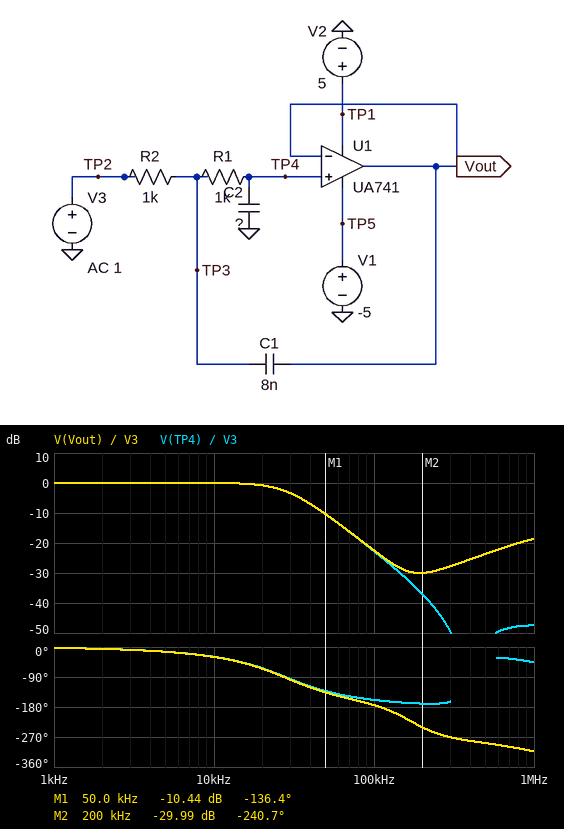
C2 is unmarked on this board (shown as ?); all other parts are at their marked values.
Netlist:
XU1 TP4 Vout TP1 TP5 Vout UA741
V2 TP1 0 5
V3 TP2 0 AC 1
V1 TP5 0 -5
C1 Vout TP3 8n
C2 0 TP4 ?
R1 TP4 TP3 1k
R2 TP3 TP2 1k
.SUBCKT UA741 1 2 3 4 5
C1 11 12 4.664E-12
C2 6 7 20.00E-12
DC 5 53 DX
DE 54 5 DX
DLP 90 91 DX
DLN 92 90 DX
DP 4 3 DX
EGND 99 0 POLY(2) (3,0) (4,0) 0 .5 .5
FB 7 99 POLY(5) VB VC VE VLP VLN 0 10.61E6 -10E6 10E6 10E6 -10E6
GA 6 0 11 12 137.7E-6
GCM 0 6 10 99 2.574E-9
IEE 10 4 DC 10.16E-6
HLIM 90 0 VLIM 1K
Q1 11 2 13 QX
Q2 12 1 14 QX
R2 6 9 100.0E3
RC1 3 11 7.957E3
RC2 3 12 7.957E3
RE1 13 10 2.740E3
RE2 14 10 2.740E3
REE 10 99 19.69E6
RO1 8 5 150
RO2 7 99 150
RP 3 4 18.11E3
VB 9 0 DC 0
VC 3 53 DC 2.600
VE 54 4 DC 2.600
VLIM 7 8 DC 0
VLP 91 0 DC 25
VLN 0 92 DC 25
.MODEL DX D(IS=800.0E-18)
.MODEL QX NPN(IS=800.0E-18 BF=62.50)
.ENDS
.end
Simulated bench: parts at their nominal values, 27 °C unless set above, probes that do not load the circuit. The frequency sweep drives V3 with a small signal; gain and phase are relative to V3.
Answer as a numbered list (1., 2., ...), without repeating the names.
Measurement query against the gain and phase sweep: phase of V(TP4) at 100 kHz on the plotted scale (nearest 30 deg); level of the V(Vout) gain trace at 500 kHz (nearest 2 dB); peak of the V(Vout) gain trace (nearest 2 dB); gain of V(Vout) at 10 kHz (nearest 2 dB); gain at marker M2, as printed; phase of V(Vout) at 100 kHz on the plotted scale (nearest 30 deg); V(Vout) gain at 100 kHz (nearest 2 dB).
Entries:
1. -150 deg
2. -24 dB
3. 0 dB
4. 0 dB
5. -29.99 dB
6. -180 deg
7. -22 dB
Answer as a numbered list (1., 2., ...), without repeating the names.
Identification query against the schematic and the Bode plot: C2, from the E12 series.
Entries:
1. 3.9 nF
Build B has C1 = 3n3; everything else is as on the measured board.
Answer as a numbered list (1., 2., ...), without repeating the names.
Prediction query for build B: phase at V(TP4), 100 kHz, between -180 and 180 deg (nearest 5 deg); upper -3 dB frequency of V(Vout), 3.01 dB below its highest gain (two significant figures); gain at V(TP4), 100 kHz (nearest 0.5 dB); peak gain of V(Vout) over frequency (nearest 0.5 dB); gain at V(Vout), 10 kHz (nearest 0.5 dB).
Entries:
1. -130 deg
2. 26 kHz
3. -16.5 dB
4. 0 dB
5. -0.5 dB
